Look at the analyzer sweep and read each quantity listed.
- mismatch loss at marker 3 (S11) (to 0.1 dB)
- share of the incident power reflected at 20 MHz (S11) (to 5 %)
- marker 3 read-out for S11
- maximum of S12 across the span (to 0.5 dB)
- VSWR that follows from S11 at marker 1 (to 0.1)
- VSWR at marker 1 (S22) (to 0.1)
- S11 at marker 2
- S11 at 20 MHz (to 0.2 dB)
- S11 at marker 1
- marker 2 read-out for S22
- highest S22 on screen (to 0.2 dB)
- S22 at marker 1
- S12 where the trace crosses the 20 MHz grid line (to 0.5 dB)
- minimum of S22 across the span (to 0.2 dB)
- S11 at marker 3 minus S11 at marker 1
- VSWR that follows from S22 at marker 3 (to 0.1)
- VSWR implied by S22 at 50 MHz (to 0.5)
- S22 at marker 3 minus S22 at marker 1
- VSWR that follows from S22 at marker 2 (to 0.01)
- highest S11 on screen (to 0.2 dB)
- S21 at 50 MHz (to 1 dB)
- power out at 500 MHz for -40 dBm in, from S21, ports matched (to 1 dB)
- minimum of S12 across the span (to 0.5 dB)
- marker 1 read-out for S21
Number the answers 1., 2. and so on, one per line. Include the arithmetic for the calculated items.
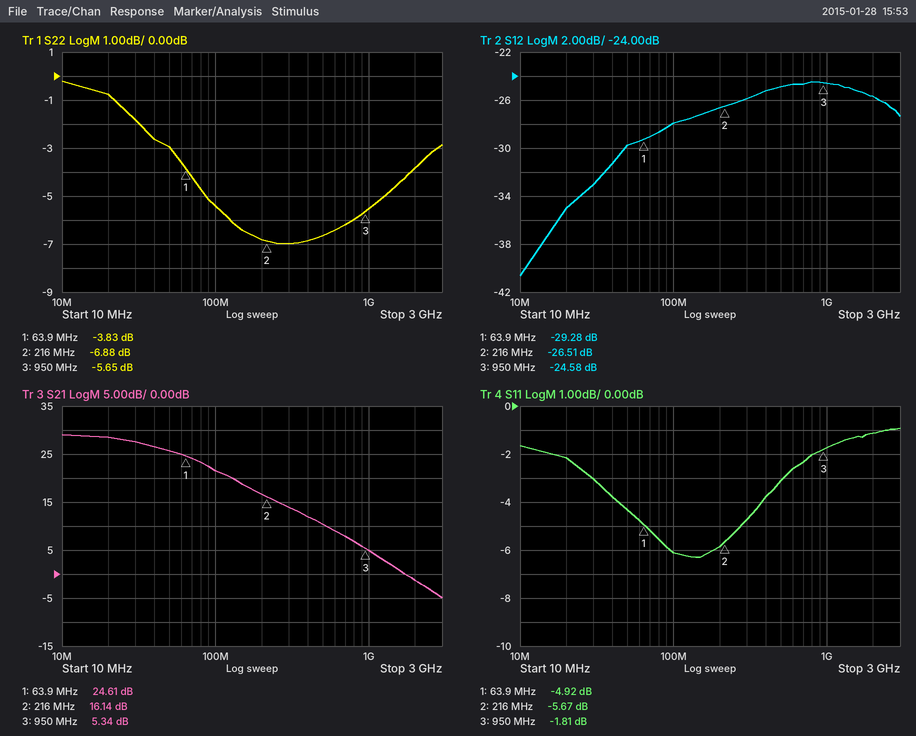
1. −10 log10(1 − 10^(-1.81/10)) ≈ 4.7 dB
2. 10^(-2.2/10) ≈ 60 %
3. -1.81 dB
4. -24.5 dB
5. (1 + 0.5675)/(1 − 0.5675) ≈ 3.6
6. (1 + 0.6434)/(1 − 0.6434) ≈ 4.6
7. -5.67 dB
8. -2.2 dB
9. -4.92 dB
10. -6.88 dB
11. -0.2 dB
12. -3.83 dB
13. -35.0 dB
14. -7.0 dB
15. -1.81 − (-4.92) = 3.11 dB
16. (1 + 0.5218)/(1 − 0.5218) ≈ 3.2
17. |Γ| = 10^(-3/20) = 0.7079; VSWR = (1 + 0.7079)/(1 − 0.7079) ≈ 5.85, so 6.0 to the nearest 0.5
18. -5.65 − (-3.83) = -1.82 dB
19. (1 + 0.4529)/(1 − 0.4529) ≈ 2.66
20. -1.0 dB
21. 26 dB
22. -40 dBm + (10 dB) = -30 dBm
23. -40.5 dB
24. 24.61 dB
